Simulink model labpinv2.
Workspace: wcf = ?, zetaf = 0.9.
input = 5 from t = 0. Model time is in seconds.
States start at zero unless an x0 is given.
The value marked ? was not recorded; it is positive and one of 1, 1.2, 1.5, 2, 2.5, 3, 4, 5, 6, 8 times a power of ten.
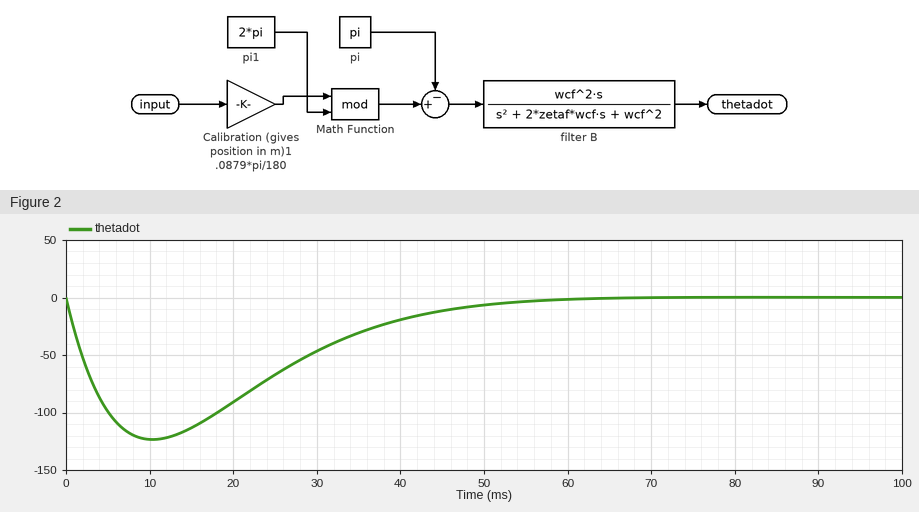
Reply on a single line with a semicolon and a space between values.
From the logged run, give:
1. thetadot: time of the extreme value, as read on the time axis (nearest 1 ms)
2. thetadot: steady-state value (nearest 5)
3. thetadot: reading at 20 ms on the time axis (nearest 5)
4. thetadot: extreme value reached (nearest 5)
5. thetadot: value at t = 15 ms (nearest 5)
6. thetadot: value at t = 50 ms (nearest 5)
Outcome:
10 ms; 0; -90; -125; -115; -5
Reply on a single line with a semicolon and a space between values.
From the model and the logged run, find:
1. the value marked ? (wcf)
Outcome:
100
